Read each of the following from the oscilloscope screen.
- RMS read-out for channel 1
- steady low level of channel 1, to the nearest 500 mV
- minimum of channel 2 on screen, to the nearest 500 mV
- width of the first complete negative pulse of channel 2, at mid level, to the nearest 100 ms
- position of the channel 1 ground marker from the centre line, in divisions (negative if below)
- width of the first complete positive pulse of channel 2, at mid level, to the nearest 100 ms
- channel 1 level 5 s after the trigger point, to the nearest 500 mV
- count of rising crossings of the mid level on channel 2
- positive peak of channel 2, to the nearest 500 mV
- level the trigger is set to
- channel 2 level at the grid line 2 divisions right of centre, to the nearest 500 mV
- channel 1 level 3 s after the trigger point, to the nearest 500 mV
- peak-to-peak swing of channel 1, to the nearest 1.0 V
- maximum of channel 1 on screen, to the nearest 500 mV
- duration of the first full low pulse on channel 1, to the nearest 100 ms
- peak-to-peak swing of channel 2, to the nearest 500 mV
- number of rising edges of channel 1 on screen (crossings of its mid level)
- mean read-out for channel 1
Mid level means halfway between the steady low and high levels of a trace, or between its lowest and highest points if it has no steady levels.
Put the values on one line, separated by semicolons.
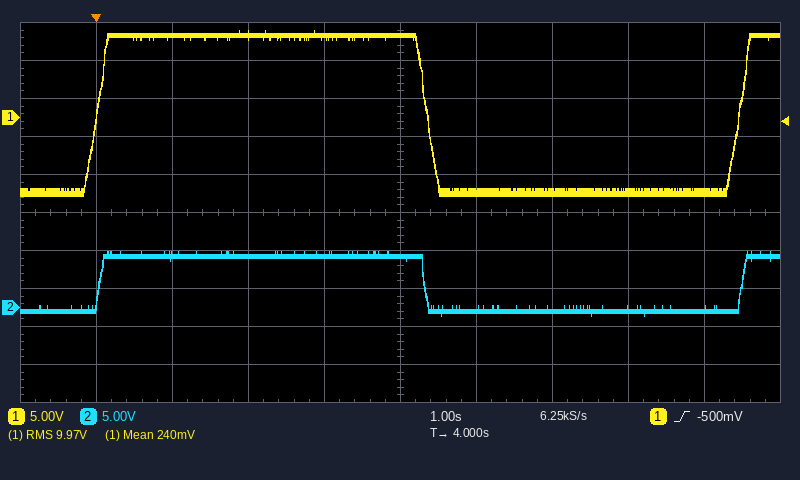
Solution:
9.97 V; -10.0 V; -1.0 V; 4.2 s; +2.5 div; 4.3 s; -10.0 V; 2; 7.5 V; -500 mV; -500 mV; 10.5 V; 22.0 V; 11.5 V; 4.1 s; 8.5 V; 2; 240 mV
